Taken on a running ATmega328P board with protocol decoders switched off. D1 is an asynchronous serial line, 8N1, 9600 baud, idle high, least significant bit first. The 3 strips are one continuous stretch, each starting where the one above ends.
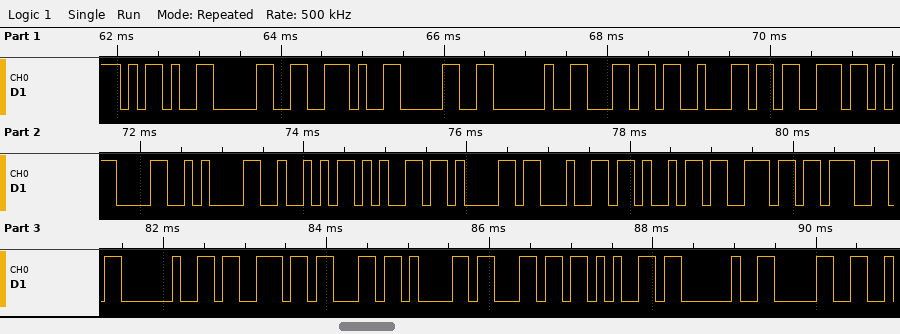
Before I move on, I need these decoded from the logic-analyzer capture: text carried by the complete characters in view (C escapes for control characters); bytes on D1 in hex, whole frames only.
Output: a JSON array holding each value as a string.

["\"-0.0 lbs\\r\\nReading scale 0\"", "0x2D 0x30 0x2E 0x30 0x20 0x6C 0x62 0x73 0x0D 0x0A 0x52 0x65 0x61 0x64 0x69 0x6E 0x67 0x20 0x73 0x63 0x61 0x6C 0x65 0x20 0x30"]
